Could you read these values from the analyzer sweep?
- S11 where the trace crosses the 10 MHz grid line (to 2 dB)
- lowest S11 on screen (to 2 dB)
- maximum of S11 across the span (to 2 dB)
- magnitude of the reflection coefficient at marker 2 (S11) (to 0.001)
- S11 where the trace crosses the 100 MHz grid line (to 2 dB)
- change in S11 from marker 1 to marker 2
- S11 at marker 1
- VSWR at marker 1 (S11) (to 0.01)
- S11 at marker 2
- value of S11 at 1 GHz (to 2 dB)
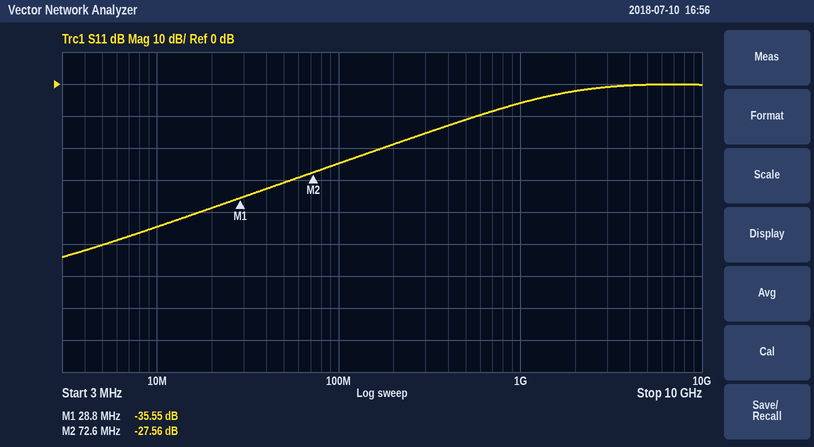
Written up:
-44 dB
-54 dB
0 dB
0.042
-24 dB
7.99 dB
-35.55 dB
1.03
-27.56 dB
-6 dB
